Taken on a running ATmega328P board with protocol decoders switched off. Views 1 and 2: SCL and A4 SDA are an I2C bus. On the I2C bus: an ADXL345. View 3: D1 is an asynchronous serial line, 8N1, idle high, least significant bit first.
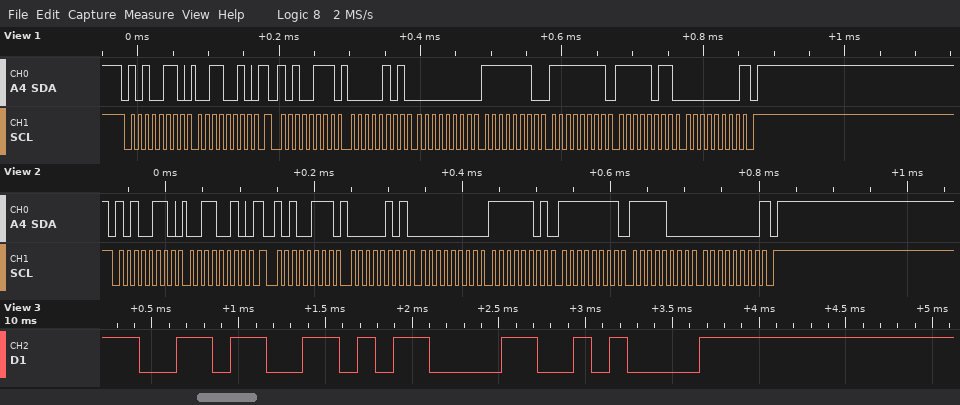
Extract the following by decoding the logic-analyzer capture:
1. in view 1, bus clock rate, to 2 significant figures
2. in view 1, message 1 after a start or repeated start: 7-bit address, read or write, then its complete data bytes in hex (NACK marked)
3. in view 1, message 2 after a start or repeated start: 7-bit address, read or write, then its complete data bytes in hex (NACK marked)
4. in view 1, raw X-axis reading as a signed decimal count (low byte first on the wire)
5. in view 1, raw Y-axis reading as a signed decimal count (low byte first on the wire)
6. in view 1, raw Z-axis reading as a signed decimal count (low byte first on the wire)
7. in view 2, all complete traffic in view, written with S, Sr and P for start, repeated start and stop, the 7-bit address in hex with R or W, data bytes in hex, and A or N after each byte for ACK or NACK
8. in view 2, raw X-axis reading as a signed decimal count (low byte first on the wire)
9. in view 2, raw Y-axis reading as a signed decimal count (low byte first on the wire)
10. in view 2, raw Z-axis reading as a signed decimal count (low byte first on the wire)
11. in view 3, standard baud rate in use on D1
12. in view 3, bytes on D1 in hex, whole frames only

100 kHz
0x53 write: 32
0x53 read: 05 00 FE FF FB 00 NACK
5
-2
251
S 53W A 32 A Sr 53R A 05 A 00 A FD A FF A F8 A 00 N P
5
-3
248
9600 baud
36 0D 0A
